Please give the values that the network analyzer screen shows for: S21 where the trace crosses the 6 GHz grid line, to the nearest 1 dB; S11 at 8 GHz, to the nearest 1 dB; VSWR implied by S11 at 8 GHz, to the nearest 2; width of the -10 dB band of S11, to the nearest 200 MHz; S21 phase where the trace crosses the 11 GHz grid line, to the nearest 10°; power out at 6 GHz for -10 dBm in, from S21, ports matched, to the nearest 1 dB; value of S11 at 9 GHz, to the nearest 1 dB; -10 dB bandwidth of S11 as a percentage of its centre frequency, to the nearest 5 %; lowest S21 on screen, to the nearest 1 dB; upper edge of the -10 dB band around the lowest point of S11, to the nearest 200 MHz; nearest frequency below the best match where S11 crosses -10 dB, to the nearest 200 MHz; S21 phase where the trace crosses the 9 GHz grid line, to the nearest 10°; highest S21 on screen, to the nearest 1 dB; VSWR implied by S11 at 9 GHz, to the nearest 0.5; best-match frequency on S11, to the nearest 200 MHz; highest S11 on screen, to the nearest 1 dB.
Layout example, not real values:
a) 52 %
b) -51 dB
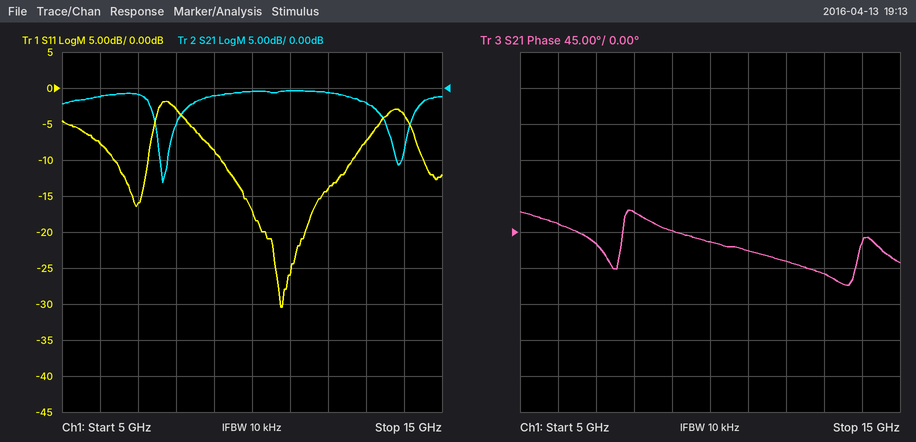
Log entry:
a) -1 dB
b) -3 dB
c) 6
d) 3.4 GHz
e) -20°
f) -11 dBm
g) -9 dB
h) 30 %
i) -13 dB
j) 12.6 GHz
k) 9.2 GHz
l) 0°
m) 0 dB
n) 2.0
o) 10.8 GHz
p) -2 dB
